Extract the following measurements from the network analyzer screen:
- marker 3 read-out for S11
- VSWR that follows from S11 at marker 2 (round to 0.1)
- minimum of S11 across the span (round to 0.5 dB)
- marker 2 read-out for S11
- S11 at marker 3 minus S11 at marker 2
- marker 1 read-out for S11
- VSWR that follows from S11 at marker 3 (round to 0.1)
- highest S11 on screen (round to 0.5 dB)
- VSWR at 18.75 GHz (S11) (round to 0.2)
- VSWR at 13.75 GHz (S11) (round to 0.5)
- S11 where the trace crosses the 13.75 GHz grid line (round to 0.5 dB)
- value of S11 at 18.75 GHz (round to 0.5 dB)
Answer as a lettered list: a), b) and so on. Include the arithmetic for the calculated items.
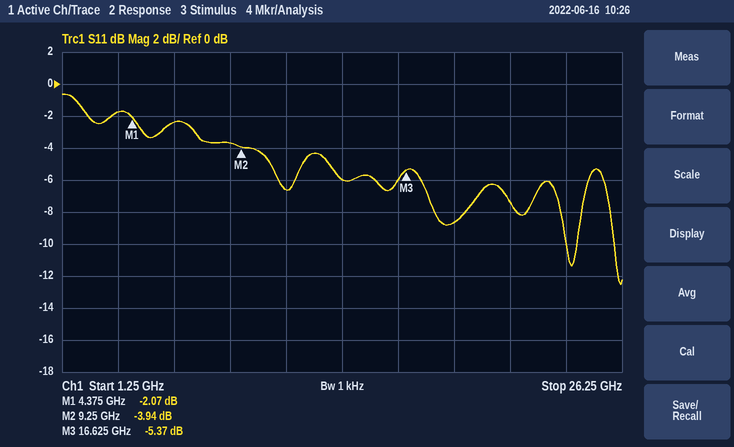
a) -5.37 dB
b) (1 + 0.6353)/(1 − 0.6353) ≈ 4.5
c) -12.5 dB
d) -3.94 dB
e) -5.37 − (-3.94) = -1.43 dB
f) -2.07 dB
g) (1 + 0.5389)/(1 − 0.5389) ≈ 3.3
h) -0.5 dB
i) |Γ| = 10^(-8.5/20) = 0.3758; VSWR = (1 + 0.3758)/(1 − 0.3758) ≈ 2.2
j) |Γ| = 10^(-6/20) = 0.5012; VSWR = (1 + 0.5012)/(1 − 0.5012) ≈ 3.0
k) -6.0 dB
l) -8.5 dB
